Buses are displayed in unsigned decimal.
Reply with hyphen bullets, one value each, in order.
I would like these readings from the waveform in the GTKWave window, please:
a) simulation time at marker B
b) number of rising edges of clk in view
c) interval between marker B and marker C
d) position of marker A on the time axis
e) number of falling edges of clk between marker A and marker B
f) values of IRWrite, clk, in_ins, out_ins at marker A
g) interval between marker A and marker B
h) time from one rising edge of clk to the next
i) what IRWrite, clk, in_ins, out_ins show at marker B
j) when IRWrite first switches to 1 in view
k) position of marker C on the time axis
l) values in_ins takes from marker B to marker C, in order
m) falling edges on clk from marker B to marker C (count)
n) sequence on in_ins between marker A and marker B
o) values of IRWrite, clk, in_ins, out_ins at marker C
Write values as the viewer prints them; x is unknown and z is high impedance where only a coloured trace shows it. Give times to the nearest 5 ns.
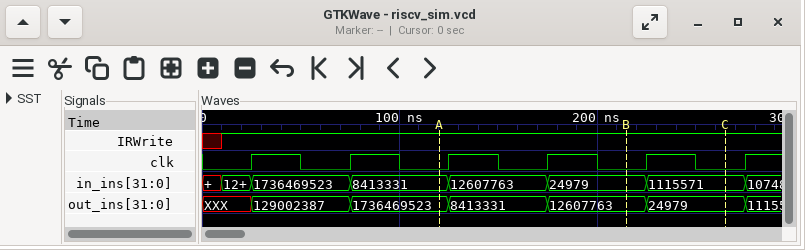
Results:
- 215 ns
- 6
- 50 ns
- 120 ns
- 2
- IRWrite=1, clk=0, in_ins=8413331, out_ins=1736469523
- 95 ns
- 50 ns
- IRWrite=1, clk=0, in_ins=24979, out_ins=12607763
- 10 ns
- 265 ns
- 24979, 1115571
- 1
- 8413331, 12607763, 24979
- IRWrite=1, clk=0, in_ins=1115571, out_ins=24979
